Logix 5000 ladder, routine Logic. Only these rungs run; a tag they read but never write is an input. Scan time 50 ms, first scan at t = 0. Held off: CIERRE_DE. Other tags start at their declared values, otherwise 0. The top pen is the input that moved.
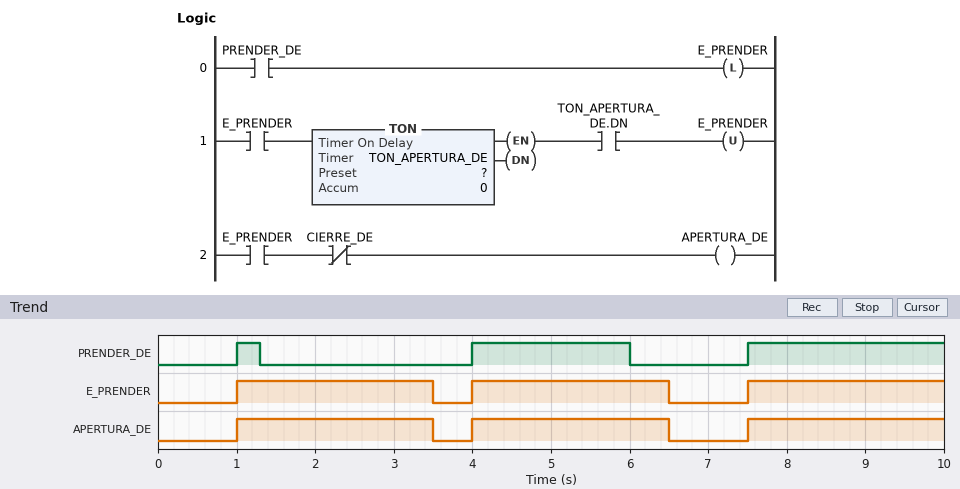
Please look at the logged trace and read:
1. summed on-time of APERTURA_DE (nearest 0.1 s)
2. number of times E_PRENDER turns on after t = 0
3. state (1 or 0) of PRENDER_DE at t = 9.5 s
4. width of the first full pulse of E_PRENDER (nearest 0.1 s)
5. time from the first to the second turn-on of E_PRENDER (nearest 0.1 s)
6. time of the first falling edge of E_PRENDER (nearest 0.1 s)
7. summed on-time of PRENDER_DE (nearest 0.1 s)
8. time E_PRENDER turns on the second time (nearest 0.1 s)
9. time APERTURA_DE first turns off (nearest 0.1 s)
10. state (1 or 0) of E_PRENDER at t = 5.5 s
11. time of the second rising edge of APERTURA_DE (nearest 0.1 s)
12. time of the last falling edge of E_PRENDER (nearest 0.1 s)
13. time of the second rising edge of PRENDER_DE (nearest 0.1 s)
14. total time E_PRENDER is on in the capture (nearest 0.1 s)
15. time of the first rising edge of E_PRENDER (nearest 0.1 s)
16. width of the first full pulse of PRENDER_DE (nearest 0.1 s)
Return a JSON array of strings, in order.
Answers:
["7.5 s", "3", "1", "2.5 s", "3.0 s", "3.5 s", "4.8 s", "4.0 s", "3.5 s", "1", "4.0 s", "6.5 s", "4.0 s", "7.5 s", "1.0 s", "0.3 s"]
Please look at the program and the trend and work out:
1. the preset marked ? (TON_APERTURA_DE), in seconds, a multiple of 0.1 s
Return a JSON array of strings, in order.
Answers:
["2.5 s"]
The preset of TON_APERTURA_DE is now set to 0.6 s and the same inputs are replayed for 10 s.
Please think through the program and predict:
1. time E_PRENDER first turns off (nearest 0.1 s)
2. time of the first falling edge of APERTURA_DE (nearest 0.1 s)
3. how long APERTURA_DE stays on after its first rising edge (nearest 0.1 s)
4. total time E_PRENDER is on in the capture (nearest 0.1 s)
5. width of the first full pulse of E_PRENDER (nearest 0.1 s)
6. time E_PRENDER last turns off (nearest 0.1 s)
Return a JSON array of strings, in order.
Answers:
["1.6 s", "1.6 s", "0.6 s", "1.8 s", "0.6 s", "8.1 s"]
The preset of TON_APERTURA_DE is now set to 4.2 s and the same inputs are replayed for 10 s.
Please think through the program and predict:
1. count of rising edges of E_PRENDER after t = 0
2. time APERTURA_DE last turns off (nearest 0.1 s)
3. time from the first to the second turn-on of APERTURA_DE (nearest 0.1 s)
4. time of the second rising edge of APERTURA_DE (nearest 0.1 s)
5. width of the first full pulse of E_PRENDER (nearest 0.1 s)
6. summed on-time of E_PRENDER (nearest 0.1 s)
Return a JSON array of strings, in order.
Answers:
["2", "5.2 s", "6.5 s", "7.5 s", "4.2 s", "6.7 s"]
